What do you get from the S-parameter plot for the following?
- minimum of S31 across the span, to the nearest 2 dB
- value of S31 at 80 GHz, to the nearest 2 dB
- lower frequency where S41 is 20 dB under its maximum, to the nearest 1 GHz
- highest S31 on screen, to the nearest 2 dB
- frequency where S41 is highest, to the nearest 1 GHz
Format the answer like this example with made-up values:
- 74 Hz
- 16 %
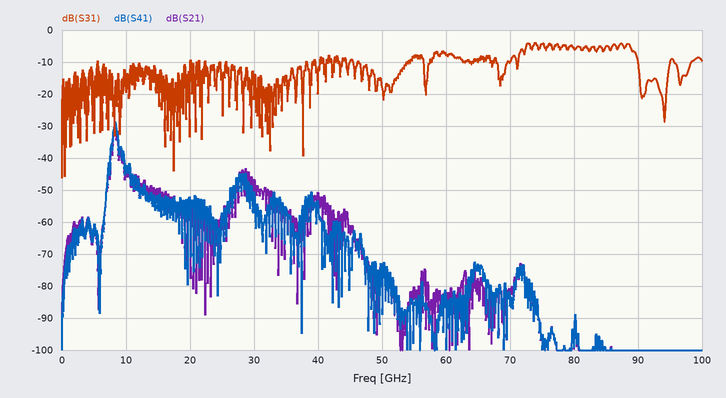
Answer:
- -46 dB
- -6 dB
- 7 GHz
- -4 dB
- 8 GHz
